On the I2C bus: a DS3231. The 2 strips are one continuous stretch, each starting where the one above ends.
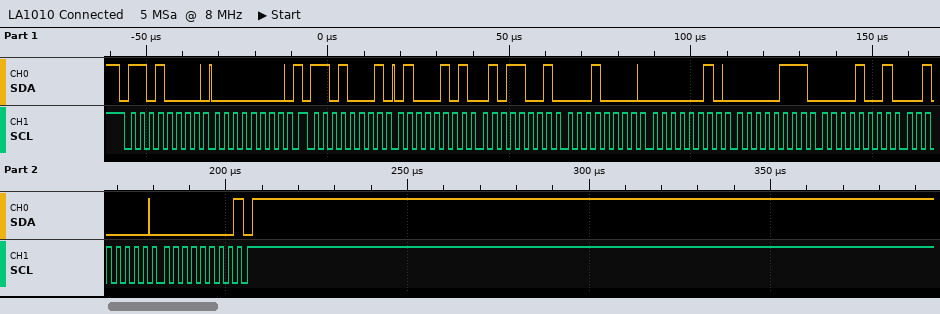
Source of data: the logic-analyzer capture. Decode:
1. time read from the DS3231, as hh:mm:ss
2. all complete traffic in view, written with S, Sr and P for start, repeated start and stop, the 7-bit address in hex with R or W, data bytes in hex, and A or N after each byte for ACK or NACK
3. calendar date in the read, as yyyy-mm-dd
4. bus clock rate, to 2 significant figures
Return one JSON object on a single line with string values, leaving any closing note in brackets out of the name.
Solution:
{"time read from the DS3231, as hh:mm:ss": "10:59:45", "all complete traffic in view, written with S, Sr and P for start, repeated start and stop, the 7-bit address in hex with R or W, data bytes in hex, and A or N after each byte for ACK or NACK": "S 68W A 00 A Sr 68R A 45 A 59 A 10 A 02 A 07 A 09 A 20 A 00 N P", "calendar date in the read, as yyyy-mm-dd": "2020-09-07", "bus clock rate, to 2 significant figures": "400 kHz"}
